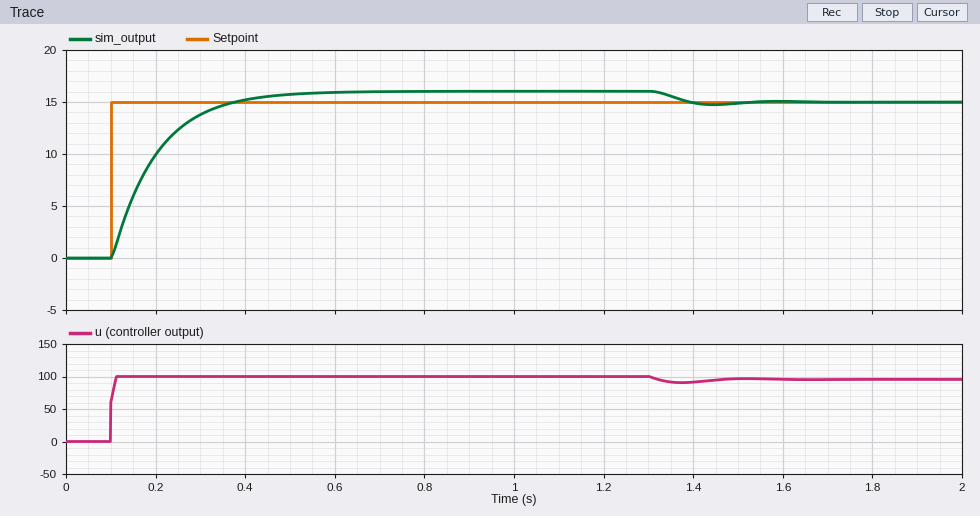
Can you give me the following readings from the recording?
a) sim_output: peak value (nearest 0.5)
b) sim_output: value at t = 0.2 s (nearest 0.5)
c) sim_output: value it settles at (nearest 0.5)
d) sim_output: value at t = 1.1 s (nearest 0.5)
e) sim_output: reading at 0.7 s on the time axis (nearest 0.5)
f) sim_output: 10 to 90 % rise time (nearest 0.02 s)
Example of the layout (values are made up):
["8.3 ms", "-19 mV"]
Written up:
["16.0", "10.0", "15.0", "16.0", "16.0", "0.18 s"]
